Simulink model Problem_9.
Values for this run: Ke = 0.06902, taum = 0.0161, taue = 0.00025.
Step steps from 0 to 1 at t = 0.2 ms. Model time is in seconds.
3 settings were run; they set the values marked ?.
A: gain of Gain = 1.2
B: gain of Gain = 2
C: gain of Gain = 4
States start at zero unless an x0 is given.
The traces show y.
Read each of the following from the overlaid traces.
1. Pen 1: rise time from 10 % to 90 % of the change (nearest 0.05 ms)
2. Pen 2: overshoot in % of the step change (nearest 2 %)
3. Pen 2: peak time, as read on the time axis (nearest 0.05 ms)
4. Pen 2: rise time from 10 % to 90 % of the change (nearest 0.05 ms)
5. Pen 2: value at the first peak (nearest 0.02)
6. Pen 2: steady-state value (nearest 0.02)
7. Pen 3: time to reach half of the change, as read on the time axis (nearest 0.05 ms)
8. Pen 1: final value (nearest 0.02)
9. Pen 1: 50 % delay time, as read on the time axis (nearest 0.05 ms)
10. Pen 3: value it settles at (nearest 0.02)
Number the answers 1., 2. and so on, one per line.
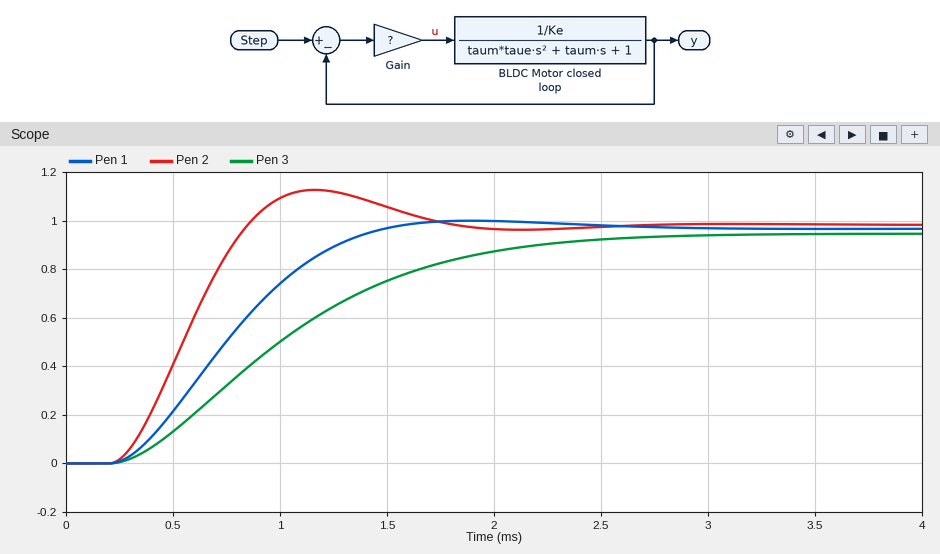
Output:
1. 0.80 ms
2. 14 %
3. 1.15 ms
4. 0.45 ms
5. 1.12
6. 0.98
7. 0.95 ms
8. 0.96
9. 0.75 ms
10. 0.94
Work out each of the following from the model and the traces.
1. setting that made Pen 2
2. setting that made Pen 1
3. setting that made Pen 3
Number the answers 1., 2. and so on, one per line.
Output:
1. C
2. B
3. A
